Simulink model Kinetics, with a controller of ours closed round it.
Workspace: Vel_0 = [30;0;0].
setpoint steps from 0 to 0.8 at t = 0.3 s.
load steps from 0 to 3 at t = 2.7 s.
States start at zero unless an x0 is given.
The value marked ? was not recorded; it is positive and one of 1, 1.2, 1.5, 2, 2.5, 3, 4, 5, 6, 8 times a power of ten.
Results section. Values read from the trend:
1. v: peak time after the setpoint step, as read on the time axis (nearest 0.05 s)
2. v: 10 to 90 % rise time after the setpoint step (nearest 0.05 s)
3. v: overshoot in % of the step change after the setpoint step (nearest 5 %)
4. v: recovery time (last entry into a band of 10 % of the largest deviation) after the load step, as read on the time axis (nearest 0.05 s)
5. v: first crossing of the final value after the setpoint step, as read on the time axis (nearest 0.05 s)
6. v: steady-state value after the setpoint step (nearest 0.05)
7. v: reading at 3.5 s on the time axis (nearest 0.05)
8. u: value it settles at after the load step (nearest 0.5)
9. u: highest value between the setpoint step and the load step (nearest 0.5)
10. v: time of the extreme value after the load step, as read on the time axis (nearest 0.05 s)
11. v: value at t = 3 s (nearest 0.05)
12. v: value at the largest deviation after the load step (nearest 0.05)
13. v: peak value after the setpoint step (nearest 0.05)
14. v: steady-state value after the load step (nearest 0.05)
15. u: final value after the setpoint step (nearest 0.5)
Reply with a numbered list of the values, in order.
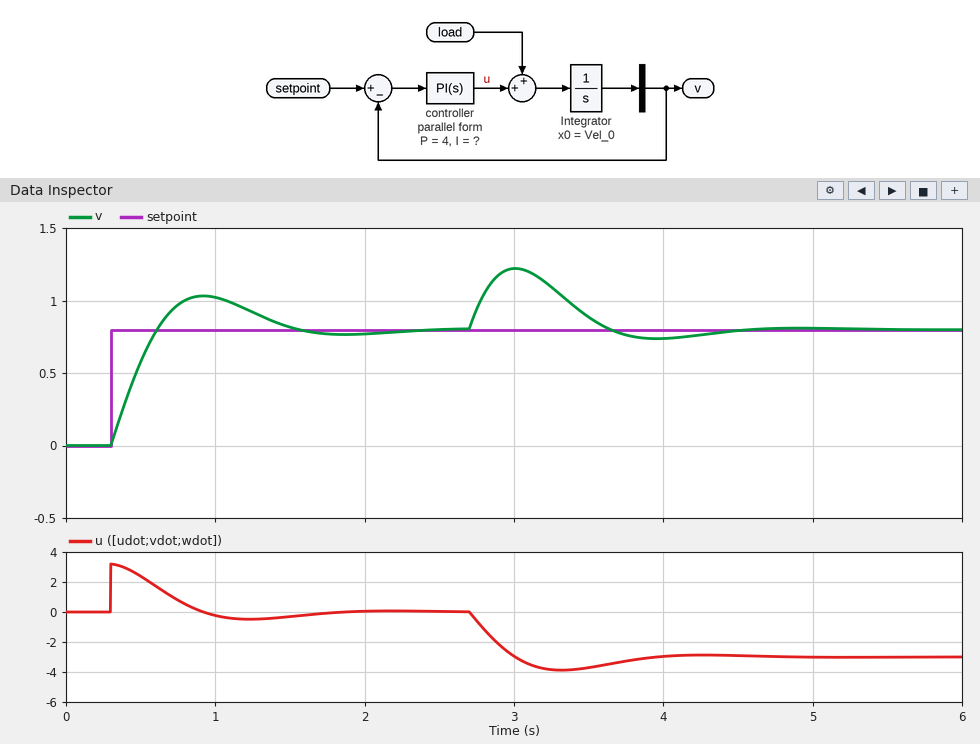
1. 0.90 s
2. 0.25 s
3. 30 %
4. 4.20 s
5. 0.60 s
6. 0.80
7. 0.90
8. -3.0
9. 3.0
10. 3.00 s
11. 1.20
12. 1.20
13. 1.05
14. 0.80
15. 0.0
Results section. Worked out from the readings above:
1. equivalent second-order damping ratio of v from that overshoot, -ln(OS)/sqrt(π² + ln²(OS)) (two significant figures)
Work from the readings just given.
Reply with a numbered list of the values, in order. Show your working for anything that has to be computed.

1. ln(0.3) = -1.204; 1.204 / sqrt(9.870 + 1.450) = 0.36
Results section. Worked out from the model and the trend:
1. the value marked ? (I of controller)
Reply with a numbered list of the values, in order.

1. 15
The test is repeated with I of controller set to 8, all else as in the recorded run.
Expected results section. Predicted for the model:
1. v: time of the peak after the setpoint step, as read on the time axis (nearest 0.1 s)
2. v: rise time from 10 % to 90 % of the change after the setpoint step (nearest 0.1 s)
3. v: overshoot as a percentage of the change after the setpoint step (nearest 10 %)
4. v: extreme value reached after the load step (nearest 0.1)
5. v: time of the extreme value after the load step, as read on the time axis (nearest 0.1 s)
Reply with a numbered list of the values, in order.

1. 1.1 s
2. 0.3 s
3. 20 %
4. 1.3
5. 3.1 s
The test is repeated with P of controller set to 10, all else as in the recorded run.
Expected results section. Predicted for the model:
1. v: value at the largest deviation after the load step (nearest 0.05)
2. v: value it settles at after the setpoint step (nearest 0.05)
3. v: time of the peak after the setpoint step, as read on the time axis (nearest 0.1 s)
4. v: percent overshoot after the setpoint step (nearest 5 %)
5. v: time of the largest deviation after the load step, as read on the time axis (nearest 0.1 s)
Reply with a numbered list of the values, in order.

1. 1.05
2. 0.80
3. 0.8 s
4. 10 %
5. 2.9 s
